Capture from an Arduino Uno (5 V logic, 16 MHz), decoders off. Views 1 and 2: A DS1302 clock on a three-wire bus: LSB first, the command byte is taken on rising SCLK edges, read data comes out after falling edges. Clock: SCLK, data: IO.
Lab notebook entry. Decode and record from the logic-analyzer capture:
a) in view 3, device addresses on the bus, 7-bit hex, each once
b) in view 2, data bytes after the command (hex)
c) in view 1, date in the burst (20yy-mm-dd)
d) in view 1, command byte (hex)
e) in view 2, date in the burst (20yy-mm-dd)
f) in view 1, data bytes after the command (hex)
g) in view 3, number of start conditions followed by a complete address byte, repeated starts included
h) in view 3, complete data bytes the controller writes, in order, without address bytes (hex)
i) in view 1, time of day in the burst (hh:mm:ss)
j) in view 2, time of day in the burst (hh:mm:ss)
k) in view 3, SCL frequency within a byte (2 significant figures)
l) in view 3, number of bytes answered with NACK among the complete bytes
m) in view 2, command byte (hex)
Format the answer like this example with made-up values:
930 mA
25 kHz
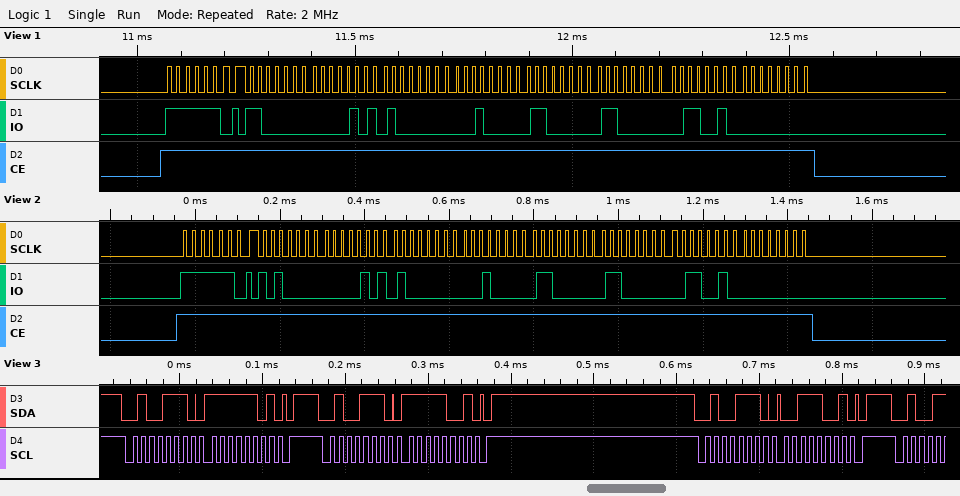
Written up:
0x27
05 50 01 04 03 03 26 00
2026-03-04
0xBF
2026-03-04
03 50 01 04 03 03 26 00
3
FD F9 39
01:50:03
01:50:05
100 kHz
0
0xBF
